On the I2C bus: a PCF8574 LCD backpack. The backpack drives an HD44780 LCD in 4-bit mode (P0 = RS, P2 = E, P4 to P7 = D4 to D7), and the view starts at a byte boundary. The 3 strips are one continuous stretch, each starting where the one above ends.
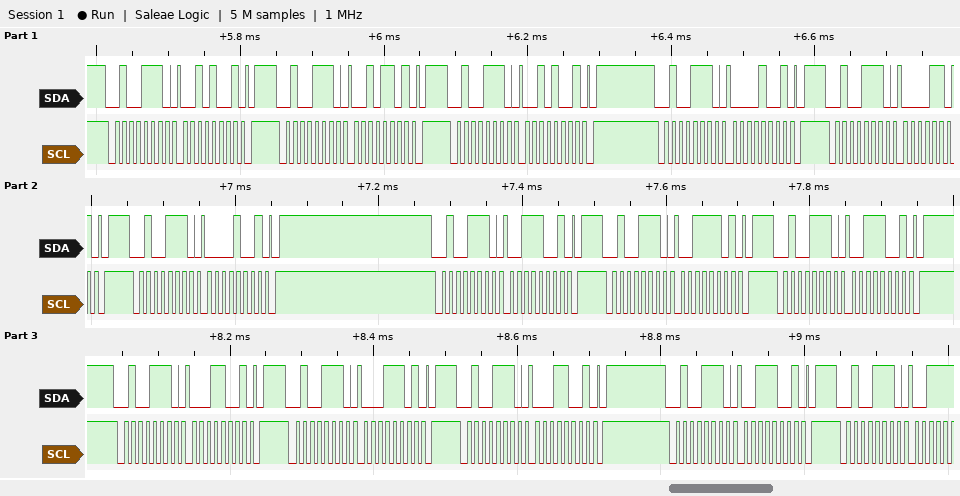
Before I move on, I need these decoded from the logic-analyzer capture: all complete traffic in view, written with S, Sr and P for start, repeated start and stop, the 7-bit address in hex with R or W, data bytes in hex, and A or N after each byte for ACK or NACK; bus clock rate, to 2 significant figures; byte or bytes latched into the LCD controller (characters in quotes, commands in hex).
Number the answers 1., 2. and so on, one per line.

1. S 27W A 29 A P S 27W A 2D A P S 27W A 29 A P S 27W A 09 A P S 27W A 0D A P S 27W A 09 A P S 27W A 39 A P S 27W A 3D A P S 27W A 39 A P S 27W A 19 A P S 27W A 1D A P S 27W A 19 A P S 27W A 39 A P S 27W A
2. 100 kHz
3. ' ' '1'
